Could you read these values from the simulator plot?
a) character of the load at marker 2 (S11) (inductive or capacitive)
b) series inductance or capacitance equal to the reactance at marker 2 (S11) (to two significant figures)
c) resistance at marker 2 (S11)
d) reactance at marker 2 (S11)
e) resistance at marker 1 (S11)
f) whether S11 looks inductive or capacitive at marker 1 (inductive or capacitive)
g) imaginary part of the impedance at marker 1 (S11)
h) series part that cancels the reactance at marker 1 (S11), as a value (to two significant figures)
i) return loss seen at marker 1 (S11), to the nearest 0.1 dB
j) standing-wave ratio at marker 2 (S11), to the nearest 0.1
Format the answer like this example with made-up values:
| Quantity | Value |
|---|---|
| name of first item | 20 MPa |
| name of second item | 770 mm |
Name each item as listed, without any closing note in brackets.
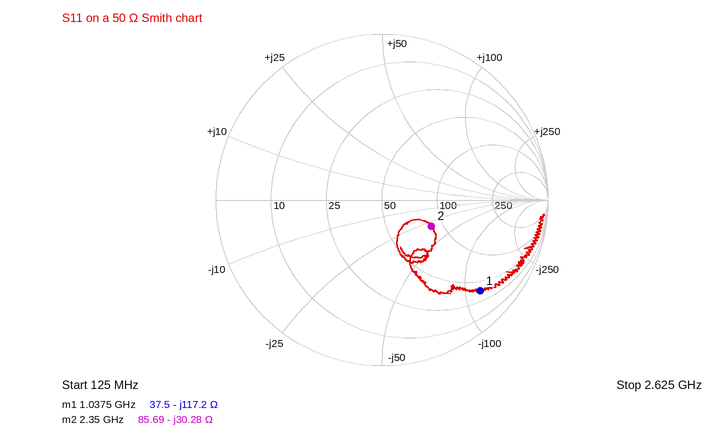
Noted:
| Quantity | Value |
|---|---|
| character of the load at marker 2 (S11) | capacitive |
| series inductance or capacitance equal to the reactance at marker 2 (S11) | 2.2 pF |
| resistance at marker 2 | 85.69 Ω |
| reactance at marker 2 | -30.28 Ω |
| resistance at marker 1 | 37.5 Ω |
| whether S11 looks inductive or capacitive at marker 1 | capacitive |
| imaginary part of the impedance at marker 1 | -117.2 Ω |
| series part that cancels the reactance at marker 1 (S11), as a value | 18 nH |
| return loss seen at marker 1 (S11), to the nearest 0.1 dB | 1.9 dB |
| standing-wave ratio at marker 2 (S11), to the nearest 0.1 | 2.0 |
